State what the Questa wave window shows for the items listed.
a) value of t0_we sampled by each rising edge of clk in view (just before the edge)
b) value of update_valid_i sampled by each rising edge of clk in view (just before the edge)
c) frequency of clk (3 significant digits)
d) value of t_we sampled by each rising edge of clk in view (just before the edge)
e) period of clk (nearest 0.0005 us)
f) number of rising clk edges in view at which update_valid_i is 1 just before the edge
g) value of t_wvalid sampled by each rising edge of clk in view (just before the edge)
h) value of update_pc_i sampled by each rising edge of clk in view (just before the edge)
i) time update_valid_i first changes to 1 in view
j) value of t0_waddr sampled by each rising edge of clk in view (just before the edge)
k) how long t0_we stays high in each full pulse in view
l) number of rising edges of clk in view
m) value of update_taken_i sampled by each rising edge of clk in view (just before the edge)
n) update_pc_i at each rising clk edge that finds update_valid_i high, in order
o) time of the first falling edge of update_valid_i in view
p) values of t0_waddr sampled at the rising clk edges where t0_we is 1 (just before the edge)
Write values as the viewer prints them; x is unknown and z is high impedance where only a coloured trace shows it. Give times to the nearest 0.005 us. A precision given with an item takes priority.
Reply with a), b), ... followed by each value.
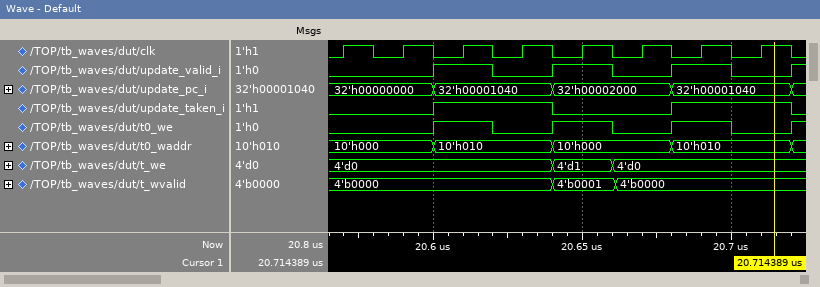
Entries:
a) 0 0 1 0 1 0 1 0
b) 0 0 1 0 1 0 1 0
c) 50.0 MHz
d) 4'd0, 4'd0, 4'd0, 4'd0, 4'd1, 4'd0, 4'd0, 4'd0
e) 0.02 us
f) 3
g) 4'b0000, 4'b0000, 4'b0000, 4'b0000, 4'b0001, 4'b0000, 4'b0000, 4'b0000
h) 32'h00000000, 32'h00000000, 32'h00001040, 32'h00001040, 32'h00002000, 32'h00002000, 32'h00001040, 32'h00001040
i) 20.6 us
j) 10'h000, 10'h000, 10'h010, 10'h010, 10'h000, 10'h000, 10'h010, 10'h010
k) 0.02 us, 0.02 us, 0.02 us
l) 8
m) 0 0 1 1 0 0 1 1
n) 32'h00001040, 32'h00002000, 32'h00001040
o) 20.62 us
p) 10'h010, 10'h000, 10'h010
